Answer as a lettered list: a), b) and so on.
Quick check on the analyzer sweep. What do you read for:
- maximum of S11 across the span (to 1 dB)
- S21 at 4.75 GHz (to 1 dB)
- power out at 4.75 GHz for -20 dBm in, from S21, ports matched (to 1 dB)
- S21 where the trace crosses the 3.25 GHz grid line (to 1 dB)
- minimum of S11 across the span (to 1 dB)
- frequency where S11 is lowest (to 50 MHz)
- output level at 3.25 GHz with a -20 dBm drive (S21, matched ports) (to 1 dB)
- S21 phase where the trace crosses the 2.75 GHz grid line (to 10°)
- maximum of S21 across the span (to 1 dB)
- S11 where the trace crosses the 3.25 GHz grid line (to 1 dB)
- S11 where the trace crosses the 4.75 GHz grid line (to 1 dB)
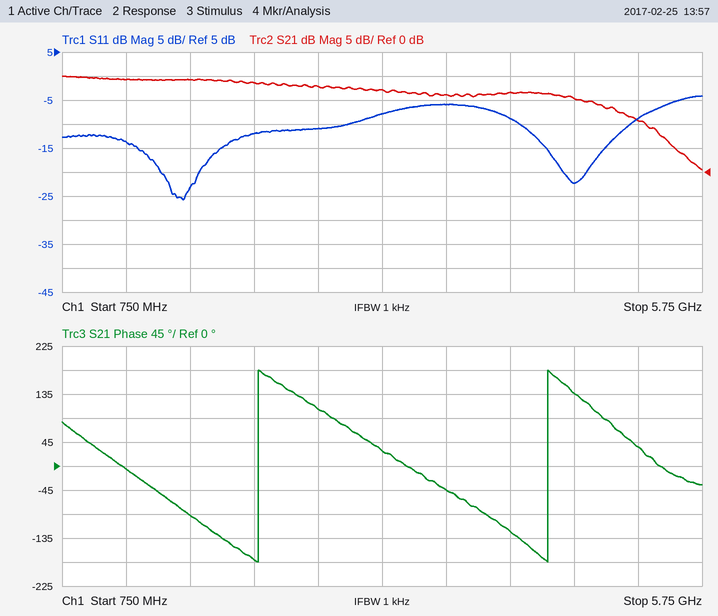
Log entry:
a) -4 dB
b) 15 dB
c) -5 dBm
d) 17 dB
e) -26 dB
f) 1.70 GHz
g) -3 dBm
h) 110°
i) 20 dB
j) -8 dB
k) -22 dB
